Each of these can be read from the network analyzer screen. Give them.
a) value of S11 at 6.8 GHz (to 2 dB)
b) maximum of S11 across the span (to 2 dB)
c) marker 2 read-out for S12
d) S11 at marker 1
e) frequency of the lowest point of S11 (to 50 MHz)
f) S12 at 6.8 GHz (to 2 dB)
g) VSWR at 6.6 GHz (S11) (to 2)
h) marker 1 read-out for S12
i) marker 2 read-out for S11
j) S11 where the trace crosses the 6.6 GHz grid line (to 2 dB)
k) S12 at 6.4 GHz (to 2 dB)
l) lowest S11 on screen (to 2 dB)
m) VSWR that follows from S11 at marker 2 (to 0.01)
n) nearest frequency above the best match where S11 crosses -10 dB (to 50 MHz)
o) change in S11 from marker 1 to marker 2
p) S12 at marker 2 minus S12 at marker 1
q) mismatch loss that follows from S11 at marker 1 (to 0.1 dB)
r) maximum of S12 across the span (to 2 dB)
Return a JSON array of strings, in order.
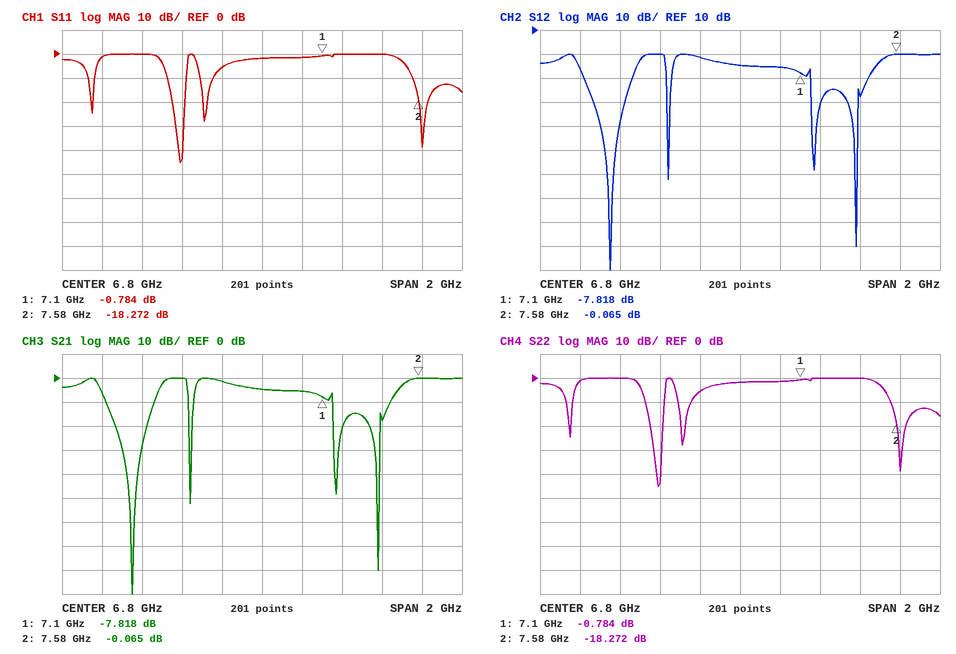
["-2 dB", "0 dB", "-0.065 dB", "-0.784 dB", "6.40 GHz", "-4 dB", "4", "-7.818 dB", "-18.272 dB", "-6 dB", "0 dB", "-46 dB", "1.28", "6.40 GHz", "-17.488 dB", "7.753 dB", "7.8 dB", "0 dB"]
